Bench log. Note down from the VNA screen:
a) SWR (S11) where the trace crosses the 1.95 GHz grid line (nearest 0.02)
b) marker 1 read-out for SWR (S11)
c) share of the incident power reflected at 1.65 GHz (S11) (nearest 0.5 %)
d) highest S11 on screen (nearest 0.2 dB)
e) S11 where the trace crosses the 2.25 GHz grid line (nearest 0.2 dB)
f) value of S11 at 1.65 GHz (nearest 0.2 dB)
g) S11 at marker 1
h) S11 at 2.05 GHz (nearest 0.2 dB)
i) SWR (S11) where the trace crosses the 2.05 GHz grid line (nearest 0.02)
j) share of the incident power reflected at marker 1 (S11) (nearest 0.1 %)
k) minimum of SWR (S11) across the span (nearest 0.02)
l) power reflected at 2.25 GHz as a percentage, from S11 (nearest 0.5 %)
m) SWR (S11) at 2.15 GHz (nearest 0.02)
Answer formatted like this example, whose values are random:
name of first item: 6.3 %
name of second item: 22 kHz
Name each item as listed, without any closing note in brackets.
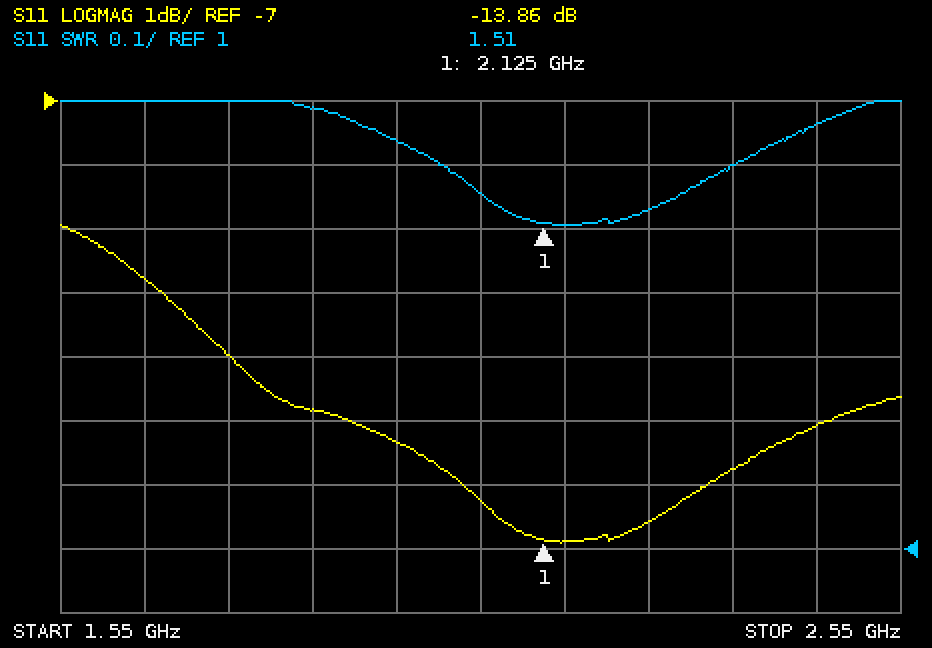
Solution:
SWR (S11) where the trace crosses the 1.95 GHz grid line: 1.64
marker 1 read-out for SWR: 1.51
share of the incident power reflected at 1.65 GHz (S11): 10.5 %
highest S11 on screen: -9.0 dB
S11 where the trace crosses the 2.25 GHz grid line: -13.6 dB
value of S11 at 1.65 GHz: -9.8 dB
S11 at marker 1: -13.86 dB
S11 at 2.05 GHz: -13.2 dB
SWR (S11) where the trace crosses the 2.05 GHz grid line: 1.56
share of the incident power reflected at marker 1 (S11): 4.1 %
minimum of SWR (S11) across the span: 1.50
power reflected at 2.25 GHz as a percentage, from S11: 4.5 %
SWR (S11) at 2.15 GHz: 1.50
